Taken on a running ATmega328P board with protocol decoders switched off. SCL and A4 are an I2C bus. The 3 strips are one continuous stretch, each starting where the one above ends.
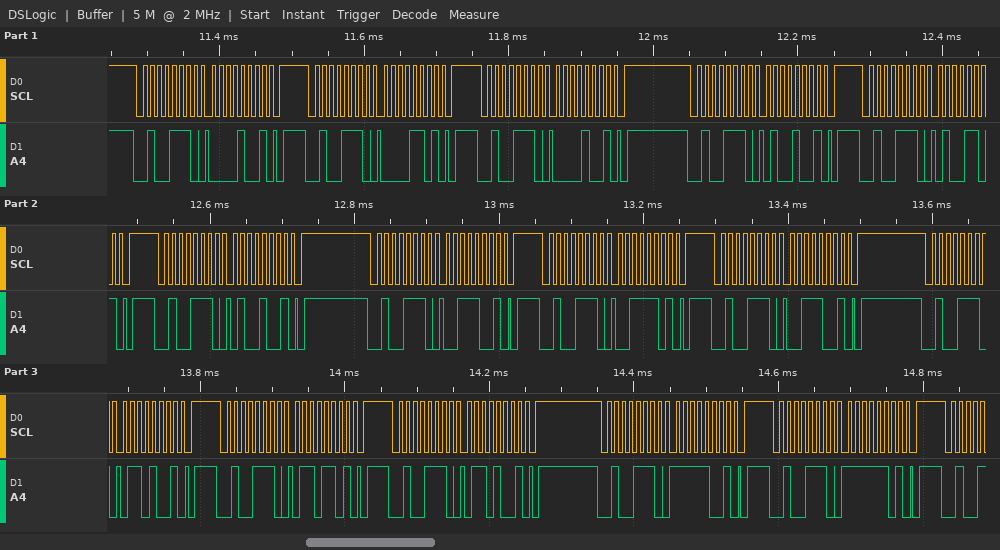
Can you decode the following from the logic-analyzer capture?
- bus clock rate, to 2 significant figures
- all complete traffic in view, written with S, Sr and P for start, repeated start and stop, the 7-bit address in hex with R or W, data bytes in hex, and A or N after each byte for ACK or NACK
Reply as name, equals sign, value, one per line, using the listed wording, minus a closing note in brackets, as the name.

bus clock rate, to 2 significant figures = 100 kHz
all complete traffic in view, written with S, Sr and P for start, repeated start and stop, the 7-bit address in hex with R or W, data bytes in hex, and A or N after each byte for ACK or NACK = S 27W A 09 A P S 27W A 0D A P S 27W A 09 A P S 27W A 49 A P S 27W A 4D A P S 27W A 49 A P S 27W A 39 A P S 27W A 3D A P S 27W A 39 A P S 27W A 69 A P S 27W A 6D A P S 27W A 69 A P S 27W A F9 A P S 27W A FD A P
